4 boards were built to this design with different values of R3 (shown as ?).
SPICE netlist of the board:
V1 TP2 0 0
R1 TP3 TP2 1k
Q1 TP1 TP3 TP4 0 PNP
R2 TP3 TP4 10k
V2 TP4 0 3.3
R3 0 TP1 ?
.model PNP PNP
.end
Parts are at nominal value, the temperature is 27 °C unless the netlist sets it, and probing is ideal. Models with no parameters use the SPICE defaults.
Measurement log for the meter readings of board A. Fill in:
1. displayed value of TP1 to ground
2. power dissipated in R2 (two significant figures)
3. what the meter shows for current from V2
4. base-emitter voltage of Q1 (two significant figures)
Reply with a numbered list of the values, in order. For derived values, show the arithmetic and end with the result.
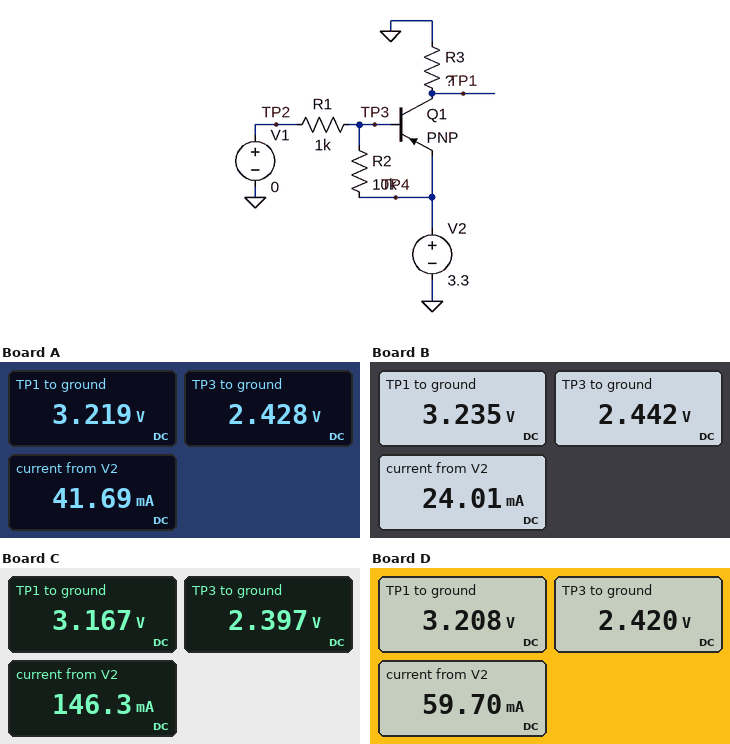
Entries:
1. 3.219 V
2. (3.3 V - 2.428 V)^2 / 10 kΩ = 76 µW
3. 41.69 mA
4. 2.428 V - 3.3 V = -870 mV
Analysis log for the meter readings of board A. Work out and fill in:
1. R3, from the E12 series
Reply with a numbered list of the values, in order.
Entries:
1. 82 Ω
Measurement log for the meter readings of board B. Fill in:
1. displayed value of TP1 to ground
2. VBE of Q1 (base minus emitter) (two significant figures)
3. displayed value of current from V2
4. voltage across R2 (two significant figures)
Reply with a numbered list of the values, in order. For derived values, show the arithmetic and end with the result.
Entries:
1. 3.235 V
2. 2.442 V - 3.3 V = -860 mV
3. 24.01 mA
4. 3.3 V - 2.442 V = 860 mV
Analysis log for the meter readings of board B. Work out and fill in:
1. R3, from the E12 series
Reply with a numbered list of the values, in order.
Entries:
1. 150 Ω
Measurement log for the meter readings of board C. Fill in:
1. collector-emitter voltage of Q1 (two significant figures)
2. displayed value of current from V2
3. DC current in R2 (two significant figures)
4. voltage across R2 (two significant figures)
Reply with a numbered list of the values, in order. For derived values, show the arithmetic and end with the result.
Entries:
1. 3.167 V - 3.3 V = -130 mV
2. 146.3 mA
3. (3.3 V - 2.397 V) / 10 kΩ = 90 µA
4. 3.3 V - 2.397 V = 900 mV
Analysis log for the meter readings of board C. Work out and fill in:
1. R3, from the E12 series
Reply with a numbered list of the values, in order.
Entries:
1. 22 Ω
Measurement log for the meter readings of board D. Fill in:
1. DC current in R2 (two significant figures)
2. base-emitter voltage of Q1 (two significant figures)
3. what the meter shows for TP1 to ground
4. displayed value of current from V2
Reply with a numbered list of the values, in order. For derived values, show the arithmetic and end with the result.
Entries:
1. (3.3 V - 2.42 V) / 10 kΩ = 88 µA
2. 2.42 V - 3.3 V = -880 mV
3. 3.208 V
4. 59.70 mA
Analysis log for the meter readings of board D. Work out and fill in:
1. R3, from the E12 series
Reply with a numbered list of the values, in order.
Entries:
1. 56 Ω
